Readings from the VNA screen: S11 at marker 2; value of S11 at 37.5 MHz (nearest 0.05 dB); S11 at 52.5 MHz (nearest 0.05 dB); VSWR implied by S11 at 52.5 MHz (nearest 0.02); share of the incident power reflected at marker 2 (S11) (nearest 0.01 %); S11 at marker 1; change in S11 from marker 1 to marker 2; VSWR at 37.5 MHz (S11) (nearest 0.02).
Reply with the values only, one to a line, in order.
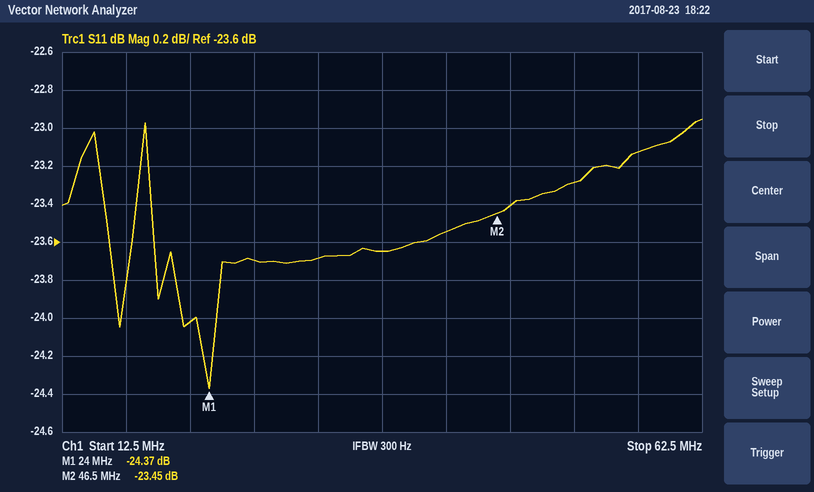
-23.45 dB
-23.65 dB
-23.30 dB
1.14
0.45 %
-24.37 dB
0.92 dB
1.14
